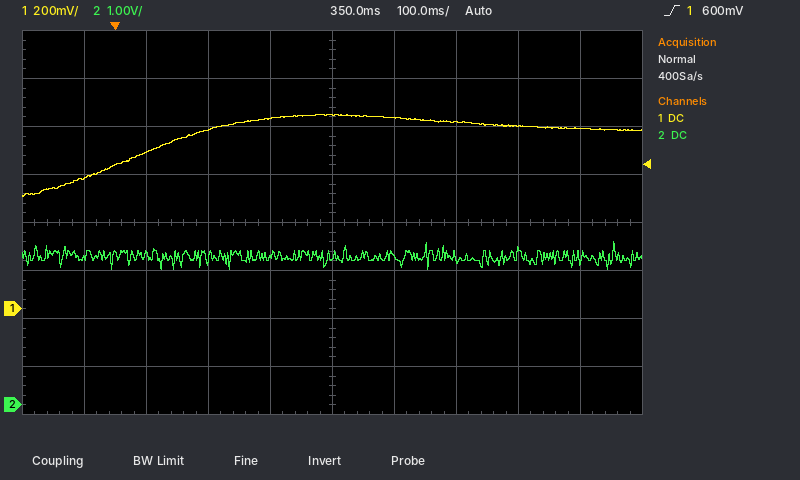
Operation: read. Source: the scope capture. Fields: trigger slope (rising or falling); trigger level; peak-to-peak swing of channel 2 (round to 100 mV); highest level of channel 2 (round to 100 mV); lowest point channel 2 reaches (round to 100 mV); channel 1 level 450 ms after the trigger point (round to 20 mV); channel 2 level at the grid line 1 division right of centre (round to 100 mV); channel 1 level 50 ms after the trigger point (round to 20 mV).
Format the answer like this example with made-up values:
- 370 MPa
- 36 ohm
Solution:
- rising
- 600 mV
- 600 mV
- 3.4 V
- 2.8 V
- 800 mV
- 3.1 V
- 660 mV
